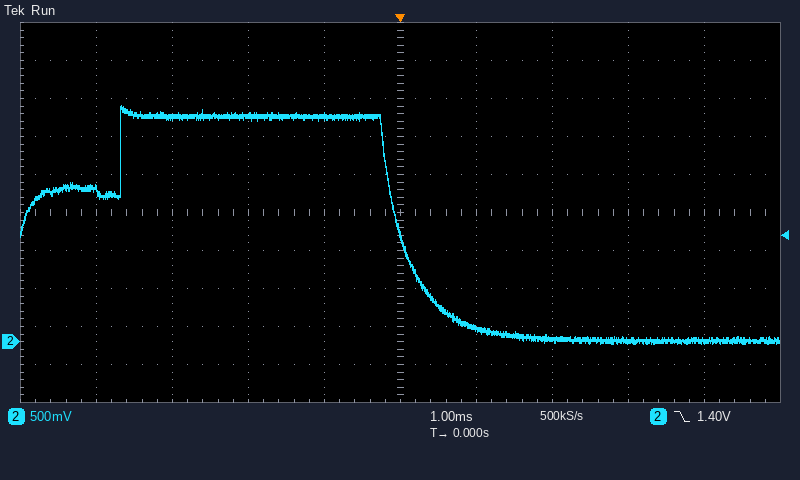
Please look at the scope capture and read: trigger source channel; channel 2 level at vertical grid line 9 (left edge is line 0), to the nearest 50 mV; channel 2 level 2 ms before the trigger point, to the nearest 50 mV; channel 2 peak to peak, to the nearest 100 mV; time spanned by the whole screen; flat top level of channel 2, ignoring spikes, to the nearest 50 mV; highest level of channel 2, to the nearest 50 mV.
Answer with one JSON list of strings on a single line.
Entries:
["channel 2", "0 mV", "2.95 V", "3.10 V", "10 ms", "2.95 V", "3.10 V"]
